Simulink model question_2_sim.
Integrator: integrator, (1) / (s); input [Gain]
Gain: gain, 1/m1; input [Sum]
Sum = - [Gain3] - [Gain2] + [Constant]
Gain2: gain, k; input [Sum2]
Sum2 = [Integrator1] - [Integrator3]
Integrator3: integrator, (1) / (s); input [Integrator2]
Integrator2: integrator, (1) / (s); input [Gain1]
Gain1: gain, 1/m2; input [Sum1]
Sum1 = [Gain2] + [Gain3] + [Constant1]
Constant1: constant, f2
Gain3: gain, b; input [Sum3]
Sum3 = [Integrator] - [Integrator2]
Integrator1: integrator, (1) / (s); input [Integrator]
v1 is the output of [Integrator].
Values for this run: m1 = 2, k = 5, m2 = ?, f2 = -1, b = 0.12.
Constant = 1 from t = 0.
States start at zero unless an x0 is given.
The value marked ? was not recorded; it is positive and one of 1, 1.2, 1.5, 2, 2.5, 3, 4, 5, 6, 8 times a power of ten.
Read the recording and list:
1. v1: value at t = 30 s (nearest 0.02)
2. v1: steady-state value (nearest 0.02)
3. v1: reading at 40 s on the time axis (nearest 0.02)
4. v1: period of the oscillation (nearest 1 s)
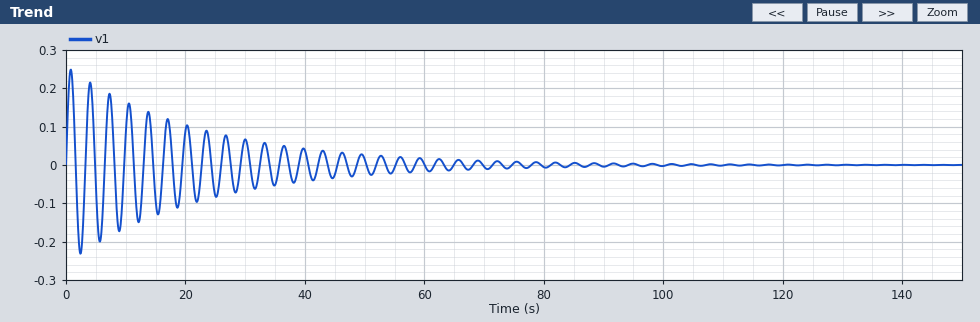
0.06
0.00
0.04
3 s
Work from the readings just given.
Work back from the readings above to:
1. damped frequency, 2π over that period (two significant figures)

2.1 rad/s
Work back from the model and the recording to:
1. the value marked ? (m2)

4
